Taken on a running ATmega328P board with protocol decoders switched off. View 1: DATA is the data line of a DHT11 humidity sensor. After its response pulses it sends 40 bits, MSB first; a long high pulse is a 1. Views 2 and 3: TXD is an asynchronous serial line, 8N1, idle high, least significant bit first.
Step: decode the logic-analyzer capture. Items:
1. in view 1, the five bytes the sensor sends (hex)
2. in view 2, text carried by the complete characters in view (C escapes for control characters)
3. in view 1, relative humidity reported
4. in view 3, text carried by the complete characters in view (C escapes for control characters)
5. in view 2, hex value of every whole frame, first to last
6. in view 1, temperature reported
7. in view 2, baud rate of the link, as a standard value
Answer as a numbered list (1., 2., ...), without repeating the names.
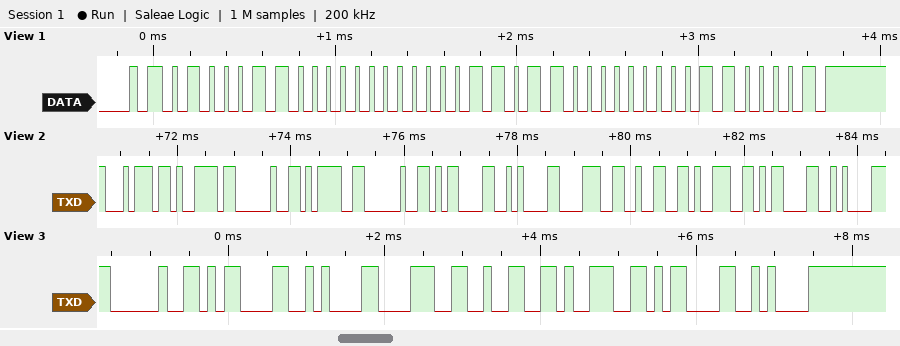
1. 46 00 1B 00 61
2. "ty = \r\n829\r\n"
3. 70 %
4. " \r\n829\r\n"
5. 74 79 20 3D 20 0D 0A 38 32 39 0D 0A
6. 27.0 °C
7. 9600 baud
